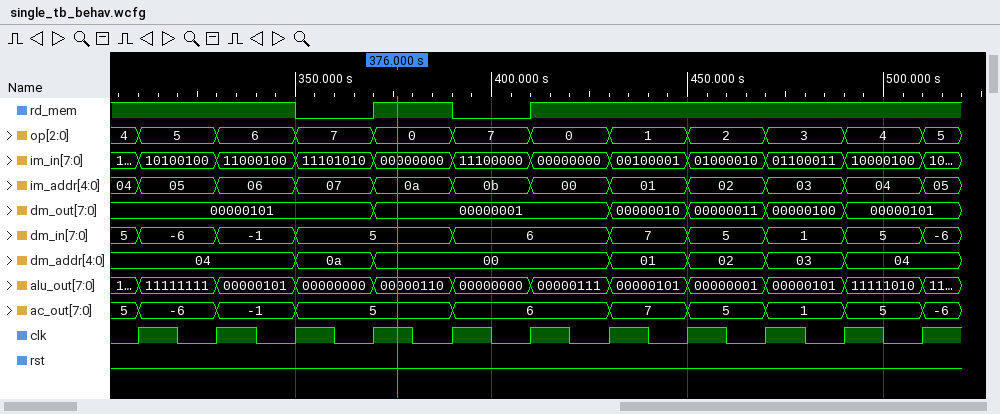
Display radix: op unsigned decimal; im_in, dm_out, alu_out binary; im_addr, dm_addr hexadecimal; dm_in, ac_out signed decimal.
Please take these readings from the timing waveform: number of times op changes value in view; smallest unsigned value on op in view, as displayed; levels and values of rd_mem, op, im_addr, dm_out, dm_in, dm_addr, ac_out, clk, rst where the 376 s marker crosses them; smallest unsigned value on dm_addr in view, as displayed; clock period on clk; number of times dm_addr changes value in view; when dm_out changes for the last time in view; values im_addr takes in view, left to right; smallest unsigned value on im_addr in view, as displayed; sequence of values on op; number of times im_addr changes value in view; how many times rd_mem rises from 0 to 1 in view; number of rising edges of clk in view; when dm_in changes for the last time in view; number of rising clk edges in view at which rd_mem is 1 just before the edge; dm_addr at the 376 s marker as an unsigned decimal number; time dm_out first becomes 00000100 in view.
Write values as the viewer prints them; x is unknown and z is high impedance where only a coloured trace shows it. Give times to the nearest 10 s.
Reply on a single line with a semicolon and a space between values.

11; 0; rd_mem=1, op=0, im_addr=0a, dm_out=00000001, dm_in=5, dm_addr=00, ac_out=5, clk=1, rst=0; 00; 20 s; 6; 490 s; 04, 05, 06, 07, 0a, 0b, 00, 01, 02, 03, 04, 05; 00; 4, 5, 6, 7, 0, 7, 0, 1, 2, 3, 4, 5; 11; 2; 11; 510 s; 9; 0; 470 s
